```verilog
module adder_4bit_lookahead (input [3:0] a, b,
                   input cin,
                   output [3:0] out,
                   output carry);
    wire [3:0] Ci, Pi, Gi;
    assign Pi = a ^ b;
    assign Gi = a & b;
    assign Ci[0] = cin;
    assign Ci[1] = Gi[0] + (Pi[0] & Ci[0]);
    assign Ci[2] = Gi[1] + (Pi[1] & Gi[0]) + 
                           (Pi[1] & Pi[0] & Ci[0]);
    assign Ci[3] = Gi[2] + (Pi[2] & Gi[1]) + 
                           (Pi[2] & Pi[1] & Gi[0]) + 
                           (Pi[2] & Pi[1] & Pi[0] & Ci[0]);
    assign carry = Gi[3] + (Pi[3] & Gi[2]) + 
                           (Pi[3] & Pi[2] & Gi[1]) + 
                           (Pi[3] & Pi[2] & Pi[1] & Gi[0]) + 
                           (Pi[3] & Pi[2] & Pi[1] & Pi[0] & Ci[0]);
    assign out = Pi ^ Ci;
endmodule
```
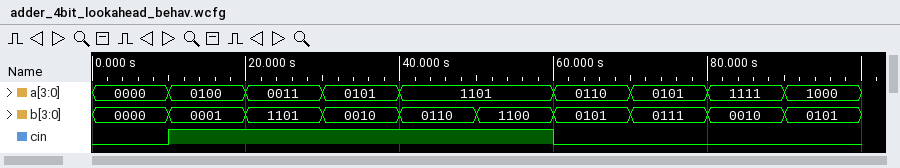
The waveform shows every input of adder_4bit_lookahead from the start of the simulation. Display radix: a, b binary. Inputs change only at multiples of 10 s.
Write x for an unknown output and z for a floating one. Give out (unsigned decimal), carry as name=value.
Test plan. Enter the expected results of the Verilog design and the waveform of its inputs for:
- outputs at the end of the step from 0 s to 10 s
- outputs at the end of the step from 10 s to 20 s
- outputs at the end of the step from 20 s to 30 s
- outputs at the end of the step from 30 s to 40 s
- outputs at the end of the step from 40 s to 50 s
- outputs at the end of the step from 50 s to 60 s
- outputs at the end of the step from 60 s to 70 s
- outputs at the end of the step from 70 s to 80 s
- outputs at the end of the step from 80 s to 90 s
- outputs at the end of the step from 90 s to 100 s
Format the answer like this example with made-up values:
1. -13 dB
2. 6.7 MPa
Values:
1. out=0, carry=0
2. out=6, carry=0
3. out=1, carry=1
4. out=8, carry=0
5. out=4, carry=1
6. out=10, carry=1
7. out=11, carry=0
8. out=12, carry=0
9. out=1, carry=1
10. out=13, carry=0
